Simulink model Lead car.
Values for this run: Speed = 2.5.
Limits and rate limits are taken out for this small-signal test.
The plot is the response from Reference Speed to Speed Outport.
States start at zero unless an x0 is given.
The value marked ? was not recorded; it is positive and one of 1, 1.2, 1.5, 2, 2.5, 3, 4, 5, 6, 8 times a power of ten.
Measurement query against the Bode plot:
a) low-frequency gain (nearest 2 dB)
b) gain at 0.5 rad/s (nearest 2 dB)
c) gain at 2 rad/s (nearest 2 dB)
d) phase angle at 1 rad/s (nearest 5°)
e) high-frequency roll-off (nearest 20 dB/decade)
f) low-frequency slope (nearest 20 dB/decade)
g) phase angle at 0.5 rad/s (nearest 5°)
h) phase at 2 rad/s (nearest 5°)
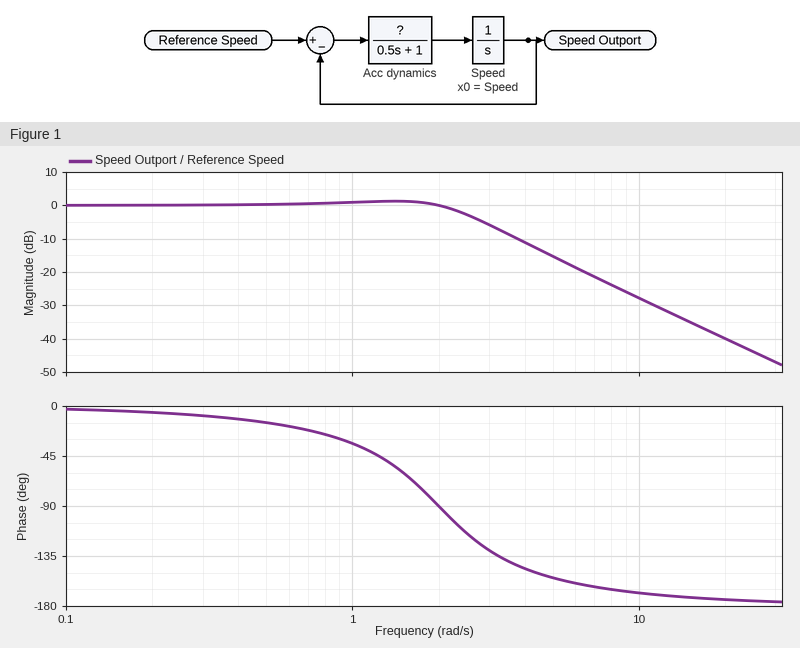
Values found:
0 dB
0 dB
0 dB
-35°
-40 dB/decade
0 dB/decade
-15°
-90°
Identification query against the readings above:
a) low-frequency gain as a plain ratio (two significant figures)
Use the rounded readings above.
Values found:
1.0
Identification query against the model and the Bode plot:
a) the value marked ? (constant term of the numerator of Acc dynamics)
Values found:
2
